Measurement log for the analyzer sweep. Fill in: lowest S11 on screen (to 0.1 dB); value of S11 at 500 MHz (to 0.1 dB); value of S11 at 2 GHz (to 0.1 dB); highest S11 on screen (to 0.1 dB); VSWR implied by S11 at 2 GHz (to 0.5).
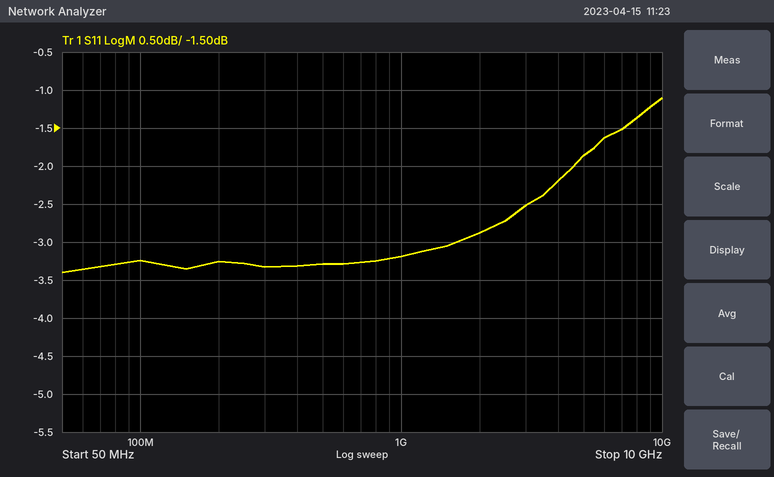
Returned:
-3.4 dB
-3.3 dB
-2.9 dB
-1.1 dB
6.0
